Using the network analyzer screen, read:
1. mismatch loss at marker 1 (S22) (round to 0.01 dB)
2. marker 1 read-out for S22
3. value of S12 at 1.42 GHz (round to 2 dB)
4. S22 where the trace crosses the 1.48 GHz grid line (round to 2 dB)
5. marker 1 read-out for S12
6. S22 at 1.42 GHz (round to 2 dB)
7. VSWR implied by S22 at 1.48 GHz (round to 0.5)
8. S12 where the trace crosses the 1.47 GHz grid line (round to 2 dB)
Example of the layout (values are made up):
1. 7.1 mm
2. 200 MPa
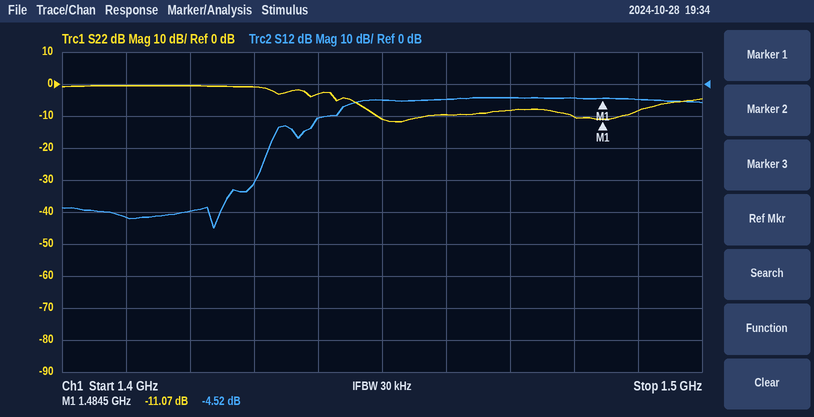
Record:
1. 0.35 dB
2. -11.07 dB
3. -40 dB
4. -10 dB
5. -4.52 dB
6. 0 dB
7. 2.0
8. -4 dB
